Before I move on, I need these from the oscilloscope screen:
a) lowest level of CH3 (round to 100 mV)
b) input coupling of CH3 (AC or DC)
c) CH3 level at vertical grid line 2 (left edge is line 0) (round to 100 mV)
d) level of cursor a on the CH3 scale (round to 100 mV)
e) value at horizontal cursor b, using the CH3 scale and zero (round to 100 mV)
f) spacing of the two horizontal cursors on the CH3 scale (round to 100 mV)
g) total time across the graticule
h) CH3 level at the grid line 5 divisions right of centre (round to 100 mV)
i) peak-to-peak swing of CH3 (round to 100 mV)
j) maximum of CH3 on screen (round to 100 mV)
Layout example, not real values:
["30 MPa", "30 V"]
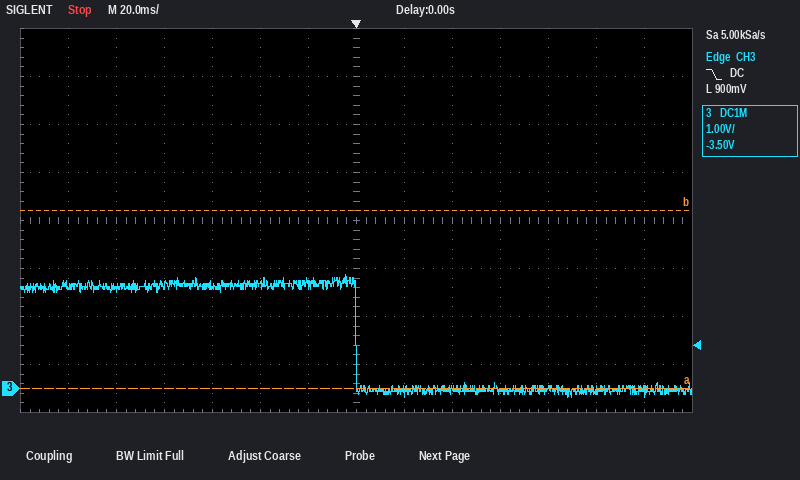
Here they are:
["-200 mV", "DC", "2.1 V", "0.0 V", "3.7 V", "3.7 V", "280 ms", "0.0 V", "2.6 V", "2.4 V"]
